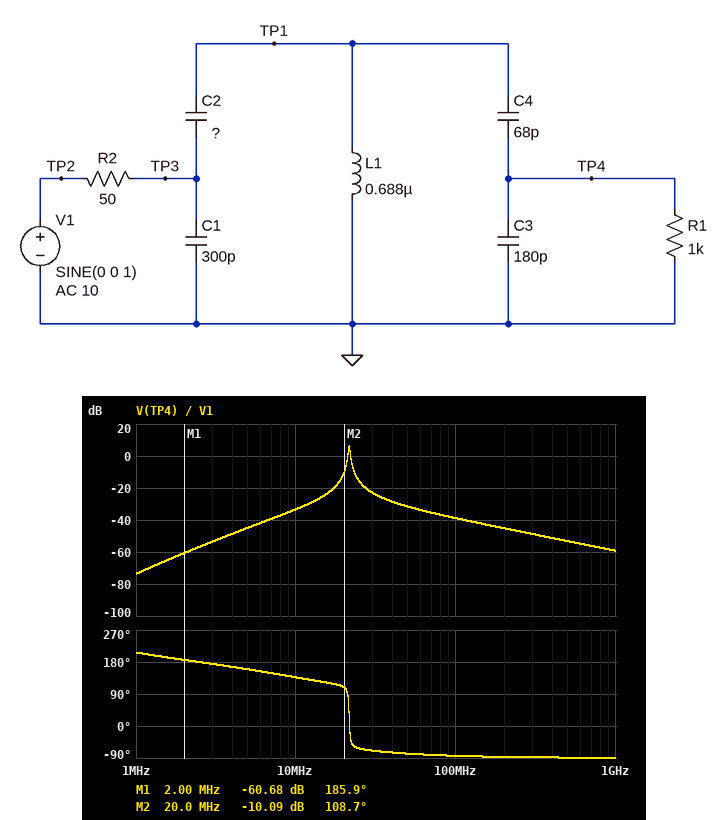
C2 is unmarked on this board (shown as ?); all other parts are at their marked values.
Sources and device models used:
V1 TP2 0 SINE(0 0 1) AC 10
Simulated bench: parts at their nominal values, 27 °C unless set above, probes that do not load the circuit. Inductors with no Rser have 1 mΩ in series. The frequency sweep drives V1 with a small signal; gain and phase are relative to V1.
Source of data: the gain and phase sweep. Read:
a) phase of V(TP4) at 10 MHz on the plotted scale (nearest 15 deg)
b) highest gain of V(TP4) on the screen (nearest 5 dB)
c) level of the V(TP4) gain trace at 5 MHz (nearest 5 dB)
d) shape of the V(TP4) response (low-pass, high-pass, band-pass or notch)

135 deg
5 dB
-45 dB
band-pass
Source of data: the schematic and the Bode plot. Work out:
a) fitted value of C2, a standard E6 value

33 pF
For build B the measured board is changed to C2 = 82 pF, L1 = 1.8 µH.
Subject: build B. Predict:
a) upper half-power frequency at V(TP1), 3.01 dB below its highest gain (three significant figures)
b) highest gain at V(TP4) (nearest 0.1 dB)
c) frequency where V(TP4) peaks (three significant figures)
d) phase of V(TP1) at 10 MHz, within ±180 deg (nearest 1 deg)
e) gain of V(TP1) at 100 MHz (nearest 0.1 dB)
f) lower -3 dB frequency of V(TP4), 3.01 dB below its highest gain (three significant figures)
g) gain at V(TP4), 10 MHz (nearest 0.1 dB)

11.3 MHz
3.1 dB
10.8 MHz
103 deg
-24.4 dB
10.4 MHz
-3.7 dB
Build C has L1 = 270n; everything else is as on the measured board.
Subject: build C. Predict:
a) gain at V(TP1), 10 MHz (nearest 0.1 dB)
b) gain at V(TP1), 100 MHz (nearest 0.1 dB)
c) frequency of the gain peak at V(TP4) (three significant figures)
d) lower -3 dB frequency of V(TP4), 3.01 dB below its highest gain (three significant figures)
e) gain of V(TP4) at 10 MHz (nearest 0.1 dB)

-31.5 dB
-26.9 dB
34.4 MHz
34.1 MHz
-42.8 dB
